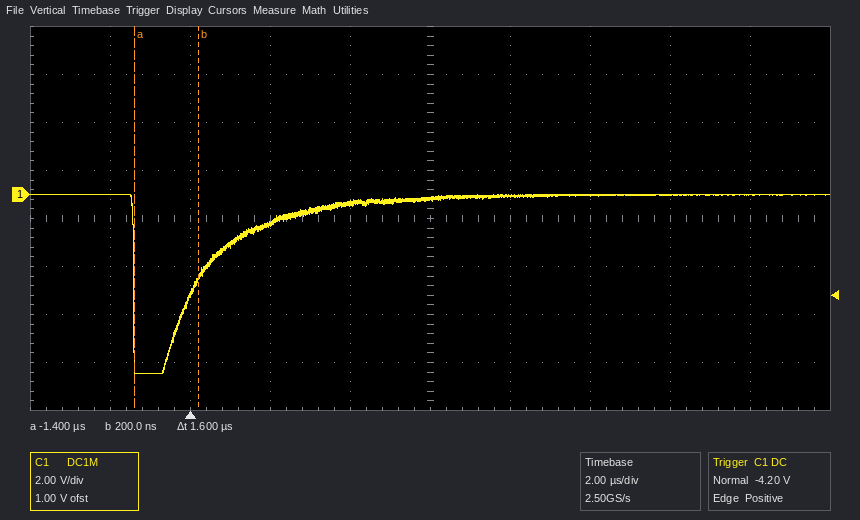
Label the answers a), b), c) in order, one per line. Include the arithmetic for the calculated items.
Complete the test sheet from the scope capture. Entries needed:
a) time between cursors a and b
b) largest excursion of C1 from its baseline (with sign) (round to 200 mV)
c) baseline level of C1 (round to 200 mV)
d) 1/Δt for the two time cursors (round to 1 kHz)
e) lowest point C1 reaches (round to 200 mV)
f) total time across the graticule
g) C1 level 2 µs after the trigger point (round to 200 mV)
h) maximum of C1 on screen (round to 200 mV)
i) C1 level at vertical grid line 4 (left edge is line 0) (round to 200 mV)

a) 1.6 µs
b) -7.4 V − (0.0 V) = -7.4 V
c) 0.0 V
d) 1 / 1.6 µs ≈ 625 kHz
e) -7.4 V
f) 20 µs
g) -1.2 V
h) 0.0 V
i) -400 mV
